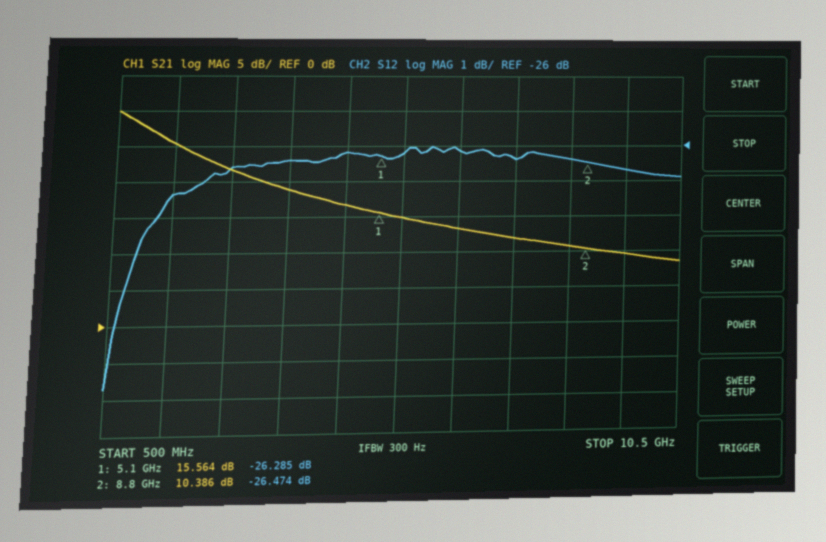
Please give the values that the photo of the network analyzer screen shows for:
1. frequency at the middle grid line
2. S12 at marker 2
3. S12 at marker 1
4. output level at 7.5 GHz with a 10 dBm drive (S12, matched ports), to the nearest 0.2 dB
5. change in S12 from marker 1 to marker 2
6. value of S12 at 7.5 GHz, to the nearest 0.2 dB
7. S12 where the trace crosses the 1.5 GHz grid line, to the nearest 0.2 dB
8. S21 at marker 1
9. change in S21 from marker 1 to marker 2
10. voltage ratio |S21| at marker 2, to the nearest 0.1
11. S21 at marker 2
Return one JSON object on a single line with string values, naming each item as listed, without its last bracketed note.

{"frequency at the middle grid line": "5.5 GHz", "S12 at marker 2": "-26.474 dB", "S12 at marker 1": "-26.285 dB", "output level at 7.5 GHz with a 10 dBm drive (S12, matched ports), to the nearest 0.2 dB": "-16.4 dBm", "change in S12 from marker 1 to marker 2": "-0.189 dB", "value of S12 at 7.5 GHz, to the nearest 0.2 dB": "-26.4 dB", "S12 where the trace crosses the 1.5 GHz grid line, to the nearest 0.2 dB": "-27.4 dB", "S21 at marker 1": "15.564 dB", "change in S21 from marker 1 to marker 2": "-5.178 dB", "voltage ratio |S21| at marker 2, to the nearest 0.1": "3.3", "S21 at marker 2": "10.386 dB"}
